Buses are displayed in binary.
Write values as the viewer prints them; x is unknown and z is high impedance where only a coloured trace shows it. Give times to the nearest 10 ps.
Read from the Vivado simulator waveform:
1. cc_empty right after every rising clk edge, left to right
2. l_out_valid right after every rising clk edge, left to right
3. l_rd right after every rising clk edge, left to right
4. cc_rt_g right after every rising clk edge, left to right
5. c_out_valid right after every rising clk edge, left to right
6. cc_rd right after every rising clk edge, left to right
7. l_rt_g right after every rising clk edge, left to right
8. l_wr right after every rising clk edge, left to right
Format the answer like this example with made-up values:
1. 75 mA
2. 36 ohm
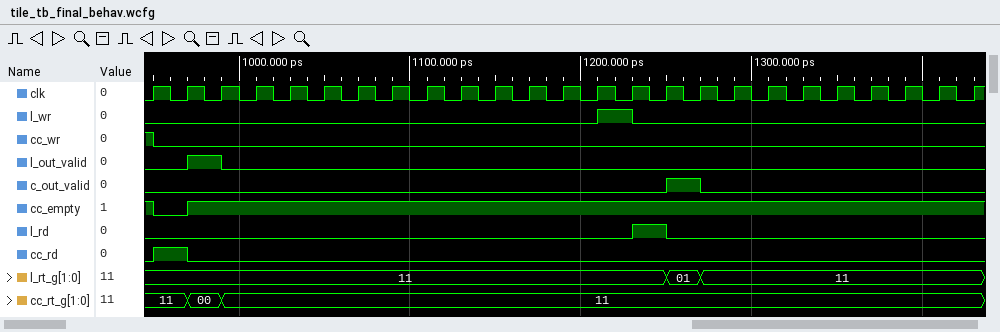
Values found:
1. 0 1 1 1 1 1 1 1 1 1 1 1 1 1 1 1 1 1 1 1 1 1 1 1 1
2. 0 1 0 0 0 0 0 0 0 0 0 0 0 0 0 0 0 0 0 0 0 0 0 0 0
3. 0 0 0 0 0 0 0 0 0 0 0 0 0 0 1 0 0 0 0 0 0 0 0 0 0
4. 11, 00, 11, 11, 11, 11, 11, 11, 11, 11, 11, 11, 11, 11, 11, 11, 11, 11, 11, 11, 11, 11, 11, 11, 11
5. 0 0 0 0 0 0 0 0 0 0 0 0 0 0 0 1 0 0 0 0 0 0 0 0 0
6. 1 0 0 0 0 0 0 0 0 0 0 0 0 0 0 0 0 0 0 0 0 0 0 0 0
7. 11, 11, 11, 11, 11, 11, 11, 11, 11, 11, 11, 11, 11, 11, 11, 01, 11, 11, 11, 11, 11, 11, 11, 11, 11
8. 0 0 0 0 0 0 0 0 0 0 0 0 0 1 0 0 0 0 0 0 0 0 0 0 0
